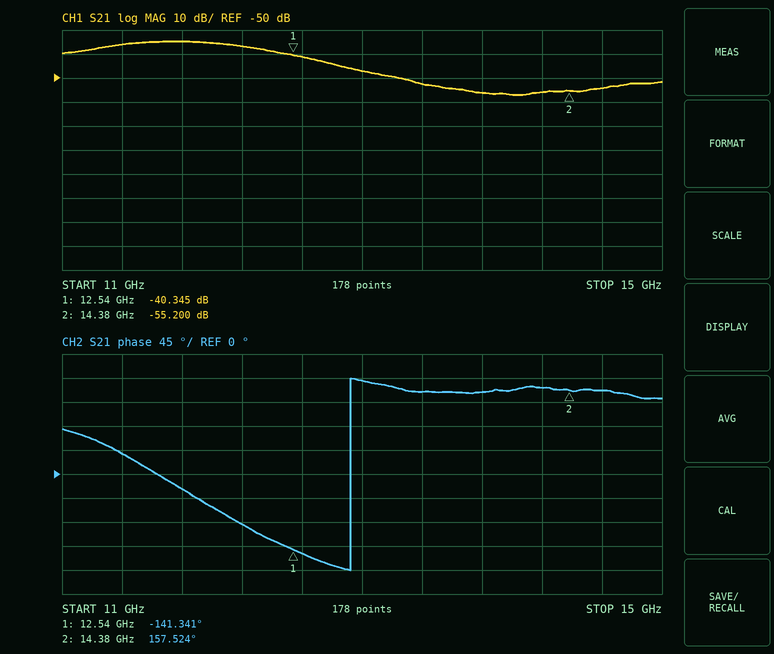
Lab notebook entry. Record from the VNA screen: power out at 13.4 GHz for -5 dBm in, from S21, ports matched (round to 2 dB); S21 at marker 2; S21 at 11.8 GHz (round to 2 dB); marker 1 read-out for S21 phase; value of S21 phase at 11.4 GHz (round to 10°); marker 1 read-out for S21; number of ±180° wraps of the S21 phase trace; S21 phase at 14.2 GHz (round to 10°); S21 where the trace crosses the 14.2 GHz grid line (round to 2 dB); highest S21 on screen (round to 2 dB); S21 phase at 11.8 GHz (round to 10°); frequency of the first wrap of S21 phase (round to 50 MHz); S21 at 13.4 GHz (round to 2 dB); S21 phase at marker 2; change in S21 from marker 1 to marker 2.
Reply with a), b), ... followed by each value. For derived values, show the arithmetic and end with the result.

a) -5 dBm + (-52 dB) = -58 dBm
b) -55.200 dB
c) -34 dB
d) -141.341°
e) 40°
f) -40.345 dB
g) 1
h) 160°
i) -56 dB
j) -34 dB
k) -30°
l) 12.90 GHz
m) -52 dB
n) 157.524°
o) -55.2 − (-40.345) = -14.855 dB
